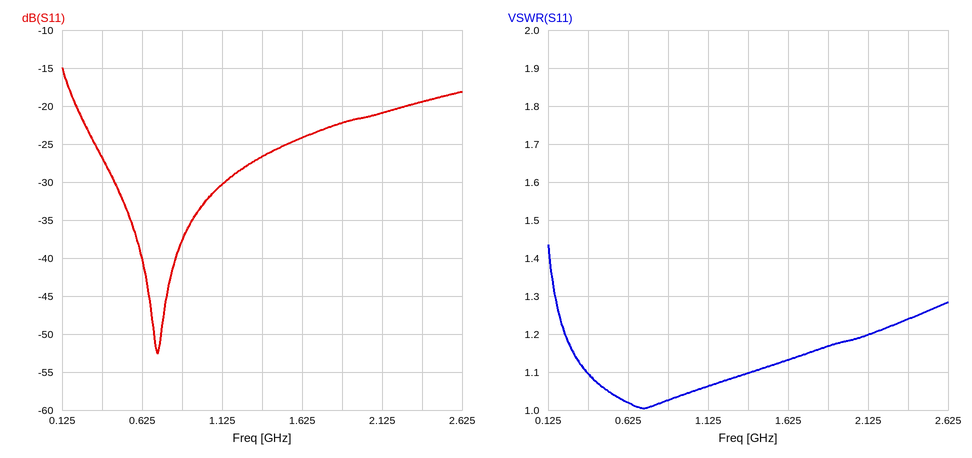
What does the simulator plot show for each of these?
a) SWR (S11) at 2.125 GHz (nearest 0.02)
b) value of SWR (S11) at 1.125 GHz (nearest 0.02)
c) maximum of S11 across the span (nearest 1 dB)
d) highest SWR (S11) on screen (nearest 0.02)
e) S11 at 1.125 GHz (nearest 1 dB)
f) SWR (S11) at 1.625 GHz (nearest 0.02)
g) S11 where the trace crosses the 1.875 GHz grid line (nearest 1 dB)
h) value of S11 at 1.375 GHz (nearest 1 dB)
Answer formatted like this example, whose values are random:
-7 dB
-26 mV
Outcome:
1.20
1.06
-15 dB
1.44
-30 dB
1.14
-22 dB
-27 dB
